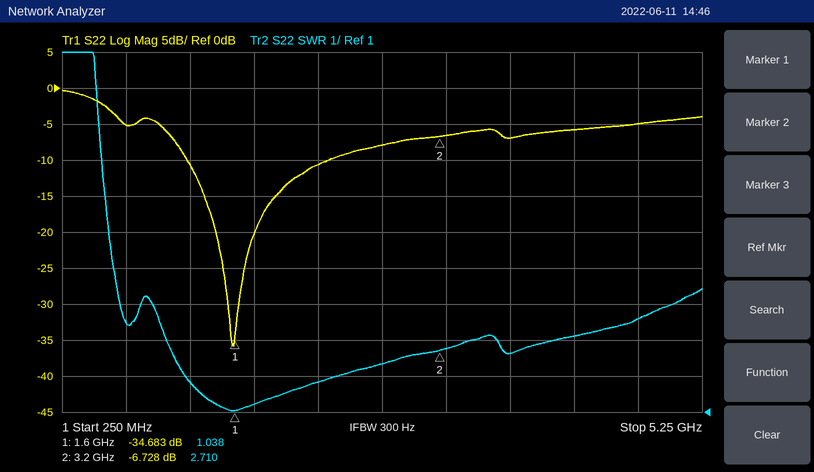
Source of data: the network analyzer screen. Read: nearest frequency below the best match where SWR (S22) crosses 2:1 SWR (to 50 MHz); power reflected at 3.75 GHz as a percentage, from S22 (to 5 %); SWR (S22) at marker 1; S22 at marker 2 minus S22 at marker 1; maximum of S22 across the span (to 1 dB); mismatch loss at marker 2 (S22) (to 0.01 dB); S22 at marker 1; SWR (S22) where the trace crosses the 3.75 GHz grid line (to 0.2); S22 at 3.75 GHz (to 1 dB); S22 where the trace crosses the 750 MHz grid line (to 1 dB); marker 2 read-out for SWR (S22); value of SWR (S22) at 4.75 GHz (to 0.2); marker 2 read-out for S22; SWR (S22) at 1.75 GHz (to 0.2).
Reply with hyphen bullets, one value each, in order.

- 1.20 GHz
- 20 %
- 1.038
- 27.955 dB
- 0 dB
- 1.04 dB
- -34.683 dB
- 2.6
- -7 dB
- -5 dB
- 2.710
- 3.6
- -6.728 dB
- 1.2
